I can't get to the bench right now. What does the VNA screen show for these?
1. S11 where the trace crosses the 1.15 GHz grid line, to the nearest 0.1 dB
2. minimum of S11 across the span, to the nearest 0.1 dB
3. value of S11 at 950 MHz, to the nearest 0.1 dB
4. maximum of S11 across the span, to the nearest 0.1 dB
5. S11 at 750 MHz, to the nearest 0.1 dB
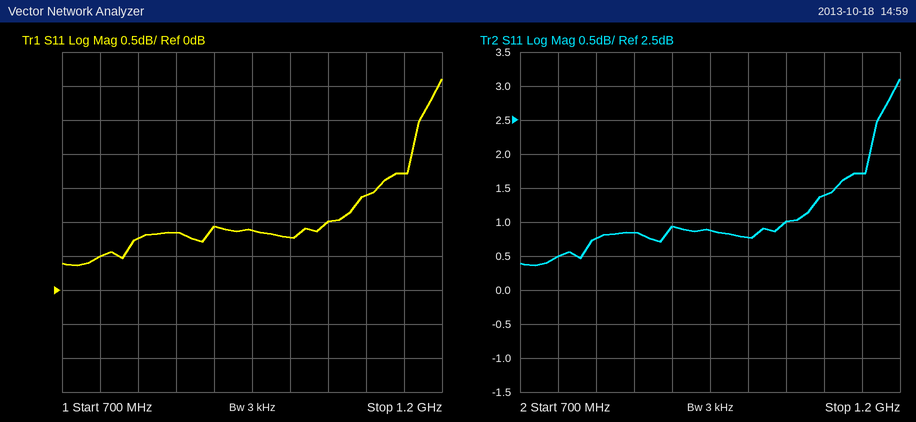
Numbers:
1.7 dB
0.4 dB
0.9 dB
3.1 dB
0.5 dB
